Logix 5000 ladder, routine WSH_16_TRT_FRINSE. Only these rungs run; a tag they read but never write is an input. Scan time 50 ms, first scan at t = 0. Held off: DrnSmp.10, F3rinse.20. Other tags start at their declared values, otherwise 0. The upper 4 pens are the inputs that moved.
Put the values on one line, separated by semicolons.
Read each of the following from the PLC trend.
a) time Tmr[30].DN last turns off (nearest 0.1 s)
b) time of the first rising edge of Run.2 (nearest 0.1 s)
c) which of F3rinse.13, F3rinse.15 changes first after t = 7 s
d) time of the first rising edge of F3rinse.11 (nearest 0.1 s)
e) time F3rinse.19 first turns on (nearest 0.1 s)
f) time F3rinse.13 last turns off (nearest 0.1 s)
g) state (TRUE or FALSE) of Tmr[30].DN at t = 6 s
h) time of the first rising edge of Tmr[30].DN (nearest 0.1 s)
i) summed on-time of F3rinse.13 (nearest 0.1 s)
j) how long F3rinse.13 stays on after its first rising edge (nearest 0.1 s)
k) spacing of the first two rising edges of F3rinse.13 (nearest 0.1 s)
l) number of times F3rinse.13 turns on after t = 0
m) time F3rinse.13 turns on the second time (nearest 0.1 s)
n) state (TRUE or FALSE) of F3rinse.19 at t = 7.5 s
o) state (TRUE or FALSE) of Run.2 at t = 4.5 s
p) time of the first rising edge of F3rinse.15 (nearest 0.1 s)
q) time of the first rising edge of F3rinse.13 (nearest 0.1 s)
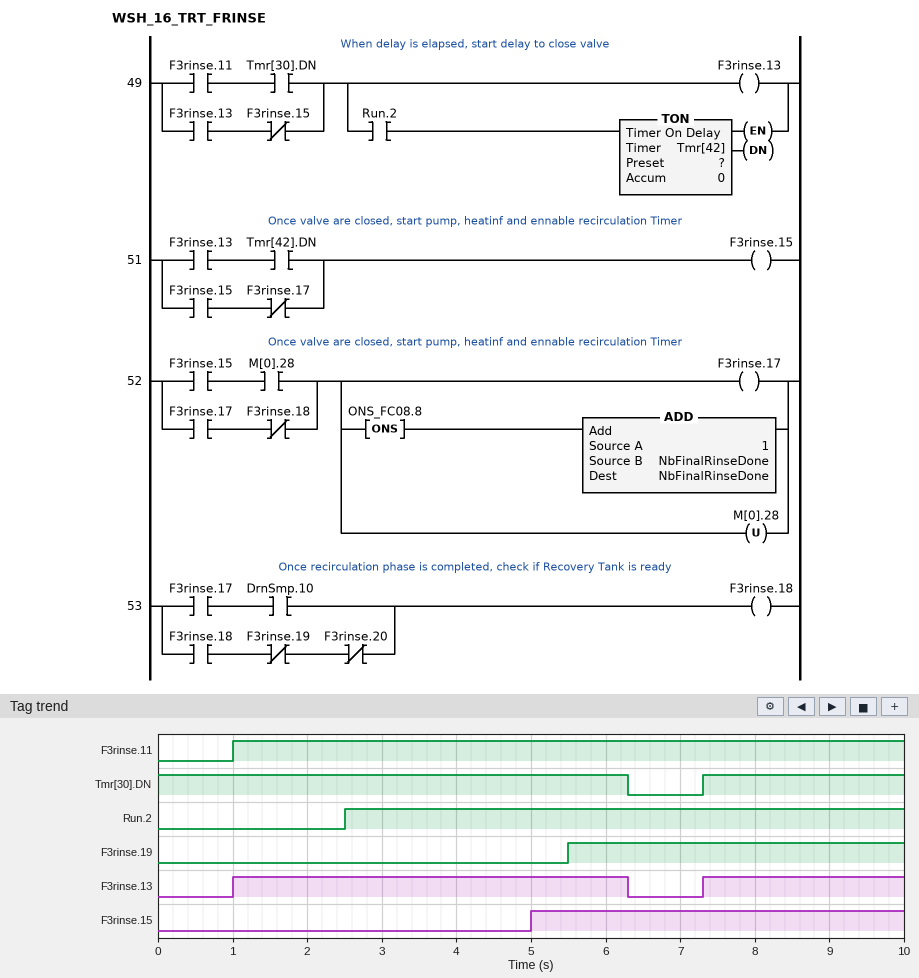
6.3 s; 2.5 s; F3rinse.13; 1.0 s; 5.5 s; 6.3 s; TRUE; 7.3 s; 8.0 s; 5.3 s; 6.3 s; 2; 7.3 s; TRUE; TRUE; 5.0 s; 1.0 s
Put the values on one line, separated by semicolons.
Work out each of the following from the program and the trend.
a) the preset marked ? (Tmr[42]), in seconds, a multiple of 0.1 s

2.5 s
